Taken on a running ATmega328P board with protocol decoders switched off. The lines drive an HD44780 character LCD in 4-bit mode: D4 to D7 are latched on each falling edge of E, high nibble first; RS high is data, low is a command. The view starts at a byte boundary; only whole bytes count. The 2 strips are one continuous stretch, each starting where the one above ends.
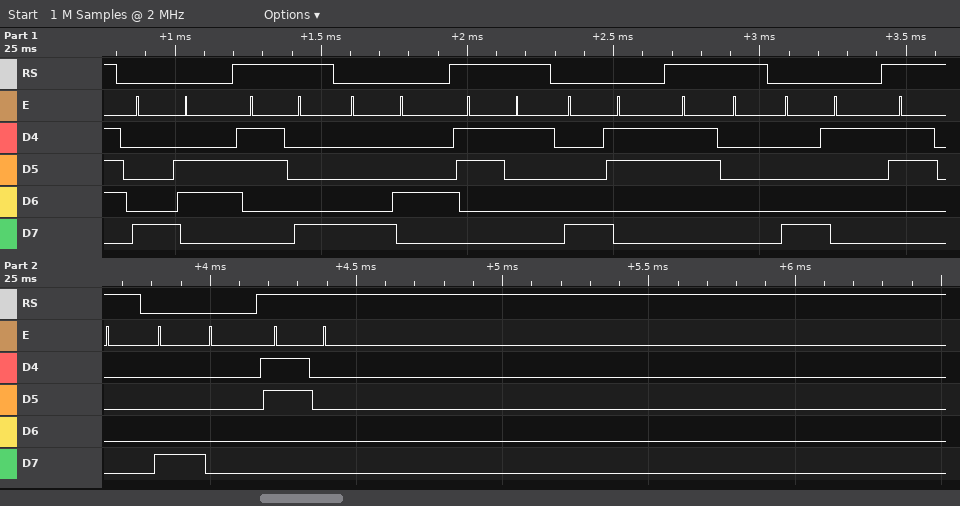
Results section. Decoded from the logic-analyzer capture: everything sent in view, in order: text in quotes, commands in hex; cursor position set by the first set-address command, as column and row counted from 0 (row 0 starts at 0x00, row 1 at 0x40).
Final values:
0x86 "8" 0x84 "1" 0x83 "0" 0x81 "0" 0x80 "0"
column 6, row 0
